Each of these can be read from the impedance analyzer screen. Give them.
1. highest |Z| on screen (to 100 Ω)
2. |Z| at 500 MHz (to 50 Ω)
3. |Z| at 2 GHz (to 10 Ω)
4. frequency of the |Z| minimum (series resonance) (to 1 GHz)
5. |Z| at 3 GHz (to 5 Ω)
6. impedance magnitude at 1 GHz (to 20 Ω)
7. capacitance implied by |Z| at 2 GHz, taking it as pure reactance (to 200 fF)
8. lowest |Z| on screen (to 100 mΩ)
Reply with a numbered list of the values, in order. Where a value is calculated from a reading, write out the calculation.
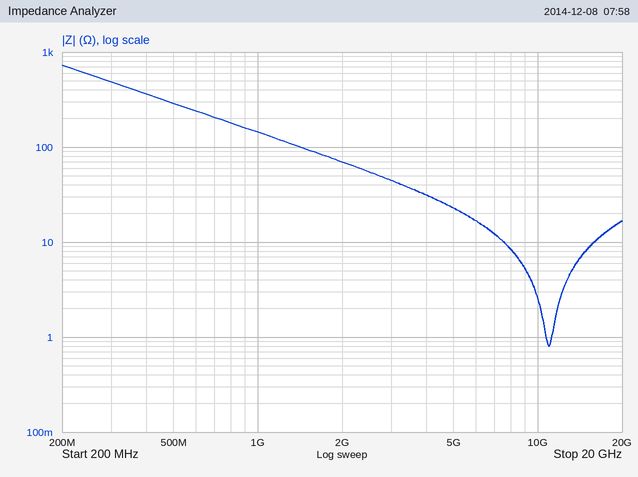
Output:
1. 700 Ω
2. 300 Ω
3. 70 Ω
4. 11 GHz
5. 45 Ω
6. 140 Ω
7. C = 1/(2π × 2 GHz × 70 Ω) ≈ 1.14 pF, so 1.2 pF to the nearest 200 fF
8. 800 mΩ
